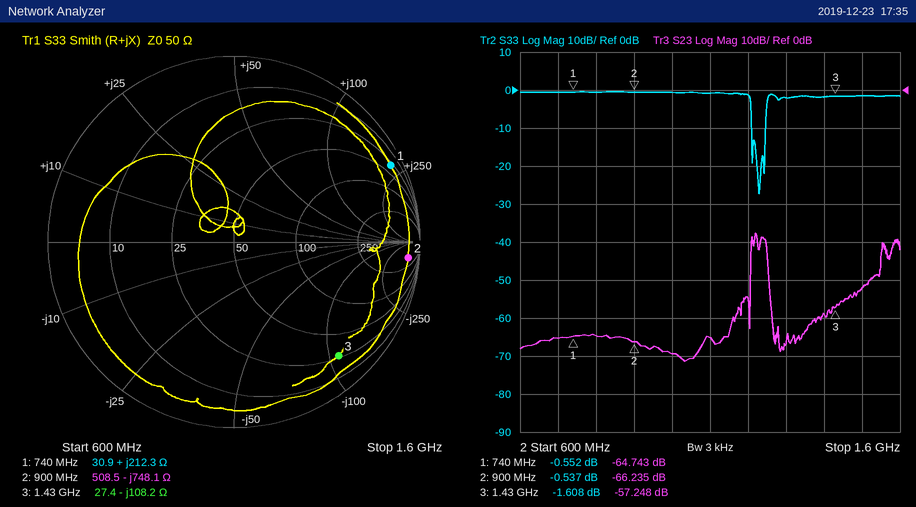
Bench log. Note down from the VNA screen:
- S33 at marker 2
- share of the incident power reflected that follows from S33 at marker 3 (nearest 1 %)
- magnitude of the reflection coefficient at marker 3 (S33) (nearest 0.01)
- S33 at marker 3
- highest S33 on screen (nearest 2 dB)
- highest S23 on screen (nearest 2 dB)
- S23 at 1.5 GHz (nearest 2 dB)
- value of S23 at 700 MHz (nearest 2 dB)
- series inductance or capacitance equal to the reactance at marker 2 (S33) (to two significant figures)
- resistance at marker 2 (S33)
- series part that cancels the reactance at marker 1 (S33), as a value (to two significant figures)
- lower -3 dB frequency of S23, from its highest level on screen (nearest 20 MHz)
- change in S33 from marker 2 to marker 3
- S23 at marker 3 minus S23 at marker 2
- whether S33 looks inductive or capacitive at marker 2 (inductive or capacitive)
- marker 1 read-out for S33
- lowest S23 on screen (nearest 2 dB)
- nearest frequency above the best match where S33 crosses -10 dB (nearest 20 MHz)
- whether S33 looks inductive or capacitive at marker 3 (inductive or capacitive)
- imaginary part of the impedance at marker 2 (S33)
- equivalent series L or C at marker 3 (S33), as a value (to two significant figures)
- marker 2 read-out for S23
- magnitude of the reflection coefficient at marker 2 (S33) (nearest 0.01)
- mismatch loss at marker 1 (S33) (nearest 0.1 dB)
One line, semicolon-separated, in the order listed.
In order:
-0.537 dB; 69 %; 0.83; -1.608 dB; 0 dB; -38 dB; -52 dB; -66 dB; 240 fF; 508.5 Ω; 1.0 pF; 1.22 GHz; -1.071 dB; 8.987 dB; capacitive; -0.552 dB; -72 dB; 1.24 GHz; capacitive; -748.1 Ω; 1.0 pF; -66.235 dB; 0.94; 9.2 dB
